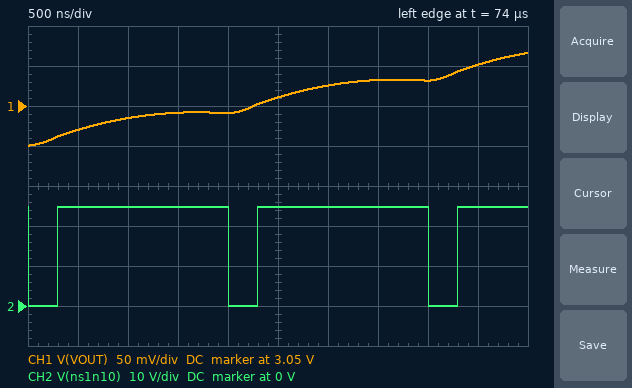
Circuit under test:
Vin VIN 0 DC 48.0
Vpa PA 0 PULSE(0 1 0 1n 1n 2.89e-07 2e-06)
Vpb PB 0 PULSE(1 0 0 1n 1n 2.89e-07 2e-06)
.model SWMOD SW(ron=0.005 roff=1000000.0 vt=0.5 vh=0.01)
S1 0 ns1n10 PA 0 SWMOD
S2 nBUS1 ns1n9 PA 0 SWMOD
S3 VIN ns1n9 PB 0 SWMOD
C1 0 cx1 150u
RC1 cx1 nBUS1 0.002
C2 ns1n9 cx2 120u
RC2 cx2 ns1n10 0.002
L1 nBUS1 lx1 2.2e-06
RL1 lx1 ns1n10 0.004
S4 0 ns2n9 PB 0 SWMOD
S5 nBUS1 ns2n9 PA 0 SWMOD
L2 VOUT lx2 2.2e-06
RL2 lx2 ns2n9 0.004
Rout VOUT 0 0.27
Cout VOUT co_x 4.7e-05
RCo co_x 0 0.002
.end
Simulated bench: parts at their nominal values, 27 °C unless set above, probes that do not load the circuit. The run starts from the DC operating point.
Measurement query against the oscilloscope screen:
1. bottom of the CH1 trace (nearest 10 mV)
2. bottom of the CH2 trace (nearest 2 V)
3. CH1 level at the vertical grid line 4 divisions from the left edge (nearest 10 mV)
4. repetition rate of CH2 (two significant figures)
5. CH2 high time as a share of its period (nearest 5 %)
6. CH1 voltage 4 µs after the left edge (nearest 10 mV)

3.00 V
0 V
3.04 V
500 kHz
85 %
3.08 V
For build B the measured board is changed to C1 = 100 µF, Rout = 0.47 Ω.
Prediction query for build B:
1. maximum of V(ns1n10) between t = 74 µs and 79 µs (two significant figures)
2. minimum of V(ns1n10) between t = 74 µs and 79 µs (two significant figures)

24 V
-6.4 mV
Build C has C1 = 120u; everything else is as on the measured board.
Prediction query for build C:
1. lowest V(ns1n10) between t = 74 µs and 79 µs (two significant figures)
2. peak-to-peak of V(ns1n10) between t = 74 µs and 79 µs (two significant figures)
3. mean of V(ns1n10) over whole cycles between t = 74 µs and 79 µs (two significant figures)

-41 mV
24 V
21 V
